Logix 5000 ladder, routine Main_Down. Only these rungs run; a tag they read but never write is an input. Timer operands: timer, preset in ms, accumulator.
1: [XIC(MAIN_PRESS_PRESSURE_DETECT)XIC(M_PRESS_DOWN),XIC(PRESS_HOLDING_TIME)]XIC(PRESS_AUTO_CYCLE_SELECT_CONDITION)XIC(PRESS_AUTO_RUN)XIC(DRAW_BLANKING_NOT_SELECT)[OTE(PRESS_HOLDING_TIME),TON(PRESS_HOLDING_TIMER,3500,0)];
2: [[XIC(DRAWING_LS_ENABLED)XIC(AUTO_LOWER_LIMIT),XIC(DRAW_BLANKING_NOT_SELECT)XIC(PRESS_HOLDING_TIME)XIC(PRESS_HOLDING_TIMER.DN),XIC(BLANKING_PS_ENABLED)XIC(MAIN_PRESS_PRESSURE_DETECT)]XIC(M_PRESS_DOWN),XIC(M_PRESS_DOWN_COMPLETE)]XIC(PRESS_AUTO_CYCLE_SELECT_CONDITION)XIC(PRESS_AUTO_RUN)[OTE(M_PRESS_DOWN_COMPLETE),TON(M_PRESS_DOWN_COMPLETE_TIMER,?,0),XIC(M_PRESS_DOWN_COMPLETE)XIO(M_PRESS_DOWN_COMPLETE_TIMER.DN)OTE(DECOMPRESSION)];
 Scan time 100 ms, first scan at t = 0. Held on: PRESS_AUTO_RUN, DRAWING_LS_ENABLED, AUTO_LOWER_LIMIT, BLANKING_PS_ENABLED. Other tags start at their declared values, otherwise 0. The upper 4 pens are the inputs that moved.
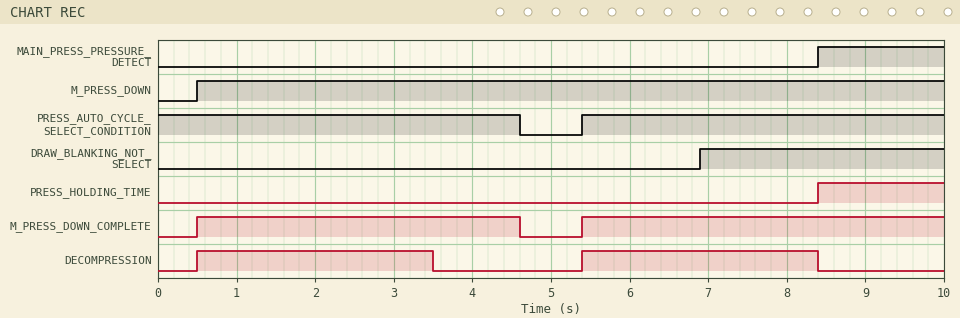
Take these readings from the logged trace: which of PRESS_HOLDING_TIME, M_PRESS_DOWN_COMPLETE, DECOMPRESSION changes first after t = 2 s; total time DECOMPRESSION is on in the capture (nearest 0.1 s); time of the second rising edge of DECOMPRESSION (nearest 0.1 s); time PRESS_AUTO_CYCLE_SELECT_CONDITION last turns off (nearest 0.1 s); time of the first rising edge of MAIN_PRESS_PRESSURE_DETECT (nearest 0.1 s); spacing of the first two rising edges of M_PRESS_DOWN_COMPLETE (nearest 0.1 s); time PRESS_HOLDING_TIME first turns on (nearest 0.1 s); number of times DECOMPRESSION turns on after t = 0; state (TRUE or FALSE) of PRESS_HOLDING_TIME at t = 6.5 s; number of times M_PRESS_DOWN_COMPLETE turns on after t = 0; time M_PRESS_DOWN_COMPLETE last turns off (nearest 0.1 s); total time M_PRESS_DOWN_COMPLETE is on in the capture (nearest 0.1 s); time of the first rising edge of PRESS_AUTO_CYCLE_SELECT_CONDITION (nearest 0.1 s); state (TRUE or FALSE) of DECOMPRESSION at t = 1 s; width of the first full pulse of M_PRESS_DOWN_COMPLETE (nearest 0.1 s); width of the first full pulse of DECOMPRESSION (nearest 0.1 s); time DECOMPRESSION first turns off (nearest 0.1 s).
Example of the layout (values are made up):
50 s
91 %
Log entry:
DECOMPRESSION
6.0 s
5.4 s
4.6 s
8.4 s
4.9 s
8.4 s
2
FALSE
2
4.6 s
8.7 s
5.4 s
TRUE
4.1 s
3.0 s
3.5 s
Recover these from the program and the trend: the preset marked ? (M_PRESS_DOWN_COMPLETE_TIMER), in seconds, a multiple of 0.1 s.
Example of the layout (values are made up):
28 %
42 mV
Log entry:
3.0 s
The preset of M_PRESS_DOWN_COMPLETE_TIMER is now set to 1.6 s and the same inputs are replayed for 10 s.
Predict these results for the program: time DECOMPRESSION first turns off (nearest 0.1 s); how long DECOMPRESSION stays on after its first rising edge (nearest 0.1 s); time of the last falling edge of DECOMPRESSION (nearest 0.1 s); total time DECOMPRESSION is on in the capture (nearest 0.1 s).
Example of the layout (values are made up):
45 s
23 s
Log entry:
2.1 s
1.6 s
7.0 s
3.2 s
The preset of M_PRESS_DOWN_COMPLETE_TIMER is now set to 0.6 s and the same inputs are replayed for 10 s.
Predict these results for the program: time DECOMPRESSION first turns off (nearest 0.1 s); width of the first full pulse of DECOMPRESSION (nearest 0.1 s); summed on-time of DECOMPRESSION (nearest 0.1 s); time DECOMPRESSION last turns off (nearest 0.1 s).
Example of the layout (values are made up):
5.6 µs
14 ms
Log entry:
1.1 s
0.6 s
1.2 s
6.0 s
